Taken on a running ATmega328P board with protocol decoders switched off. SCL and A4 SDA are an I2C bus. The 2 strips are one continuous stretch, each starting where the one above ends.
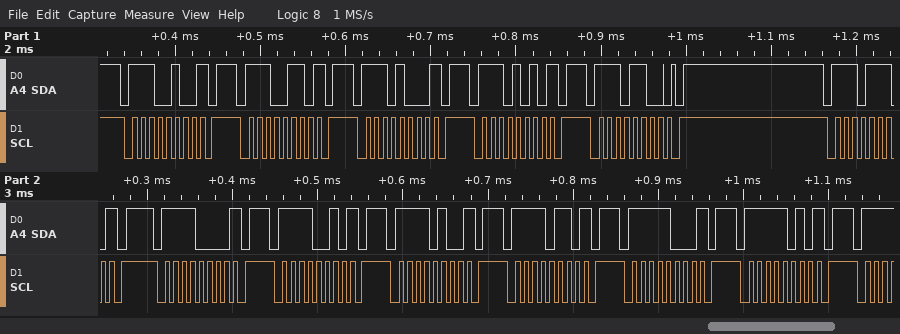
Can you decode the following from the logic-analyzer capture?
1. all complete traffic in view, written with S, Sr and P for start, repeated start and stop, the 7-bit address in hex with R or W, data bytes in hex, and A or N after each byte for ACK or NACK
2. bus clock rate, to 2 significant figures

S 72W N P S 73W N P S 74W N P S 75W N P S 76W A P S 77W N P S 78W N P S 79W N P S 7AW N P S 7BW N P S 7CW N P S 7DW N P
100 kHz
